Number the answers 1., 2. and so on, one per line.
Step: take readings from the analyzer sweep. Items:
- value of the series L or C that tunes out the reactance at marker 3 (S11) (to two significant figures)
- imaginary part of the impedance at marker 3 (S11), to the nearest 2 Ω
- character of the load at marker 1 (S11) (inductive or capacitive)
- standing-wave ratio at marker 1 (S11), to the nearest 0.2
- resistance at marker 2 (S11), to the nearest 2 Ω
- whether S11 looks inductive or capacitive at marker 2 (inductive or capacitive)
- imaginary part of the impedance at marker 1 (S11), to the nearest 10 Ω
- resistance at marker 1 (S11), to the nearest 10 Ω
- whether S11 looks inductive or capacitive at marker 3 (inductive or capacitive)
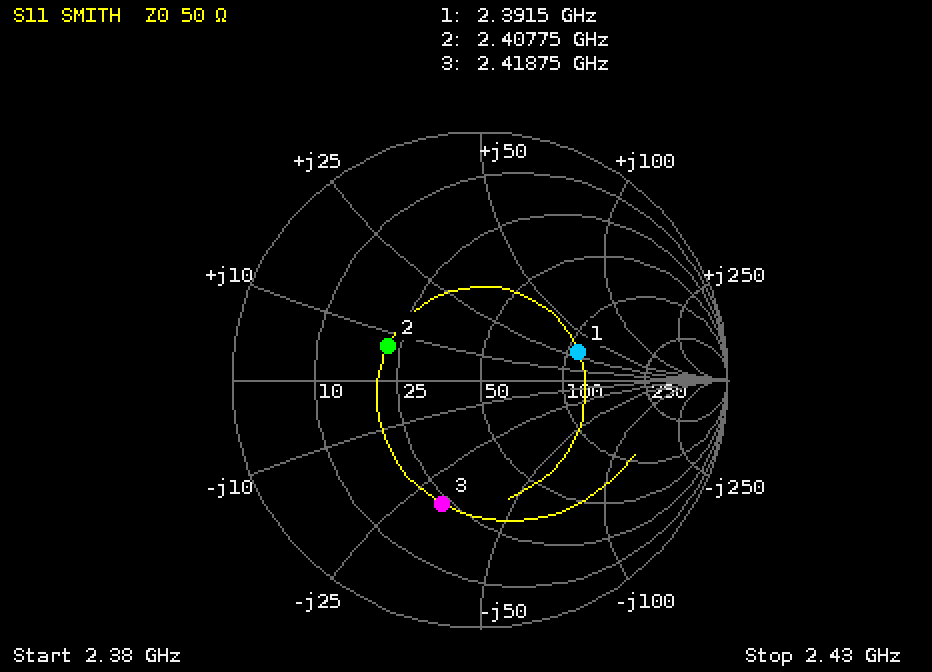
1. 2.1 nH
2. -32 Ω
3. inductive
4. 2.4
5. 22 Ω
6. inductive
7. +30 Ω
8. 110 Ω
9. capacitive
